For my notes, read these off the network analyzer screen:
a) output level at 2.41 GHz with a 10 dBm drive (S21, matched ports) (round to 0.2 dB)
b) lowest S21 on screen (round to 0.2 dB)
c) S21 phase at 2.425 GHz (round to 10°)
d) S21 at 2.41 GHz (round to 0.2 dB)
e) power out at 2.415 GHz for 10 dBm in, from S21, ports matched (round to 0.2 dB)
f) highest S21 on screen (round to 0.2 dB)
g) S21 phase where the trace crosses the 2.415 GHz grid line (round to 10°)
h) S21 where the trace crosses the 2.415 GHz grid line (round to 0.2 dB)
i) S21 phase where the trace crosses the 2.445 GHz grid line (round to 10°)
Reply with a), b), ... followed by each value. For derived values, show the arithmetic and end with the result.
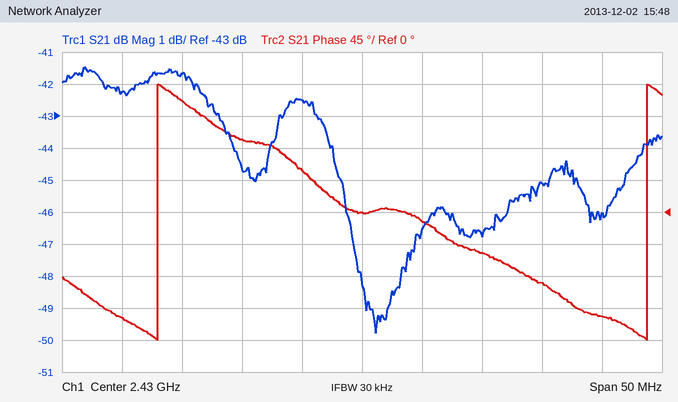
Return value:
a) 10 dBm + (-42.2 dB) = -32.2 dBm
b) -49.8 dB
c) 60°
d) -42.2 dB
e) 10 dBm + (-41.6 dB) = -31.6 dBm
f) -41.4 dB
g) 160°
h) -41.6 dB
i) -100°
